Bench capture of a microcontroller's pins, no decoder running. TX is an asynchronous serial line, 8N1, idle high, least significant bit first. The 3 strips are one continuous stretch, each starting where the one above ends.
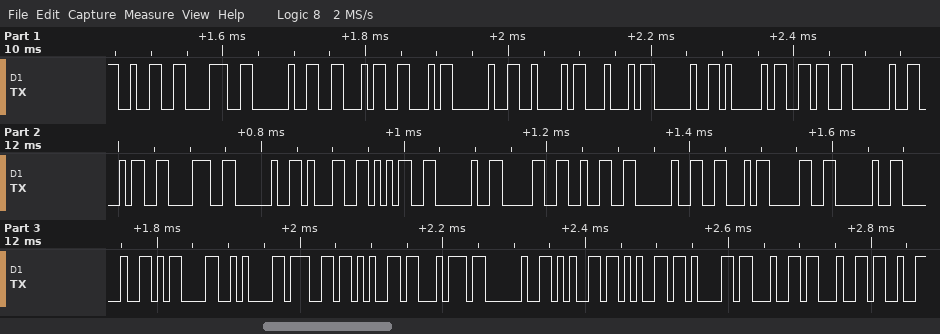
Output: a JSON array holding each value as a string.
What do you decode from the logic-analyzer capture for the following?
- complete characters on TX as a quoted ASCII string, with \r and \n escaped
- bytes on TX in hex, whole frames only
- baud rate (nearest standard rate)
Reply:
["\"28 FF BD A6 48 15 02 F0  \\r\\nget eeadd\"", "32 38 20 46 46 20 42 44 20 41 36 20 34 38 20 31 35 20 30 32 20 46 30 20 20 0D 0A 67 65 74 20 65 65 61 64 64", "115200 baud"]
